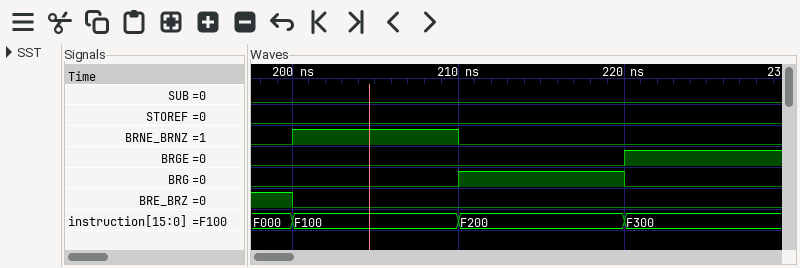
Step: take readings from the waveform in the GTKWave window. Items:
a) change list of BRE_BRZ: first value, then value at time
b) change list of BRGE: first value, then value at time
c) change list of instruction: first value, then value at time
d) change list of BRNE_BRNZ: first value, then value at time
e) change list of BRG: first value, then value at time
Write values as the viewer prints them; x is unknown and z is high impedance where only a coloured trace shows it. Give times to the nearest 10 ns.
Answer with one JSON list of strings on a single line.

["1, 0 at 200 ns", "0, 1 at 220 ns", "F000, F100 at 200 ns, F200 at 210 ns, F300 at 220 ns", "0, 1 at 200 ns, 0 at 210 ns", "0, 1 at 210 ns, 0 at 220 ns"]
